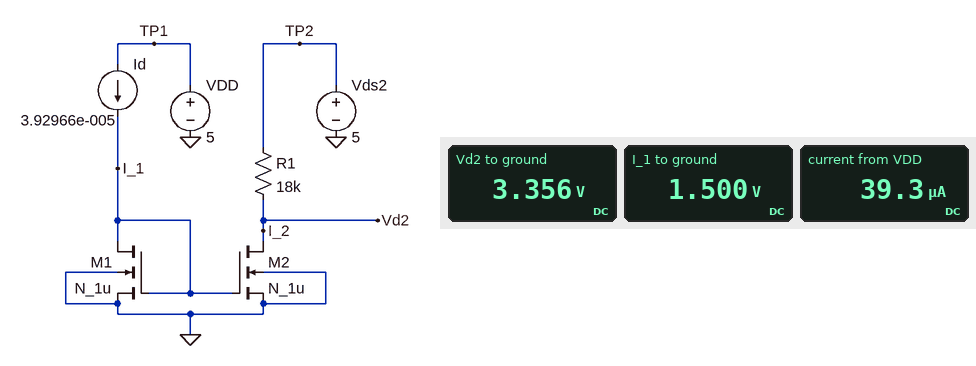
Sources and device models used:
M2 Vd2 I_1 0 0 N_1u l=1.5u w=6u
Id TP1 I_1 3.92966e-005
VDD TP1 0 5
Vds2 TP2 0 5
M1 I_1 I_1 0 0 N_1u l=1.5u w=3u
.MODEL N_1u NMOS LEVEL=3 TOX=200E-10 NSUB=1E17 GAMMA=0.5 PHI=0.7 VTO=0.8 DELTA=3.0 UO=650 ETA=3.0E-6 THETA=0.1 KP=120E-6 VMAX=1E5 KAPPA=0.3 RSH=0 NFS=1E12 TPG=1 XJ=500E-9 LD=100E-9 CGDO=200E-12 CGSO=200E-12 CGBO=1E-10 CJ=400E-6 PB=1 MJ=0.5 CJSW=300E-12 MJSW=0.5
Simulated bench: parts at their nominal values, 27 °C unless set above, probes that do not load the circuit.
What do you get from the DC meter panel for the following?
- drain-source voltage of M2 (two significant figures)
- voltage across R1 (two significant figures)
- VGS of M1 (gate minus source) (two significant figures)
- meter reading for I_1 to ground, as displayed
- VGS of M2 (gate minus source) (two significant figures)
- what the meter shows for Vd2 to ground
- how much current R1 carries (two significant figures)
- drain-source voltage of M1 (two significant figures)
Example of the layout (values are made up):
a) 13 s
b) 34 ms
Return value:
a) 3.4 V
b) 1.6 V
c) 1.5 V
d) 1.500 V
e) 1.5 V
f) 3.356 V
g) 91 µA
h) 1.5 V
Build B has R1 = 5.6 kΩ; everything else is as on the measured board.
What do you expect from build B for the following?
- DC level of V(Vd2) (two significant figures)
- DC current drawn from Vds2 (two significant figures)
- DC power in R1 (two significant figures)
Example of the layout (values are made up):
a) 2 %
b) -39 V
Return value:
a) 4.5 V
b) 93 µA
c) 48 µW
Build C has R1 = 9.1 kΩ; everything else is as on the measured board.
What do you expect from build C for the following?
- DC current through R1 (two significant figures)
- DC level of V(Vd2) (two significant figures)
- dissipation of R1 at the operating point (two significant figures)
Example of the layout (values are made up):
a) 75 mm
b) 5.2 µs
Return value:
a) 92 µA
b) 4.2 V
c) 78 µW
